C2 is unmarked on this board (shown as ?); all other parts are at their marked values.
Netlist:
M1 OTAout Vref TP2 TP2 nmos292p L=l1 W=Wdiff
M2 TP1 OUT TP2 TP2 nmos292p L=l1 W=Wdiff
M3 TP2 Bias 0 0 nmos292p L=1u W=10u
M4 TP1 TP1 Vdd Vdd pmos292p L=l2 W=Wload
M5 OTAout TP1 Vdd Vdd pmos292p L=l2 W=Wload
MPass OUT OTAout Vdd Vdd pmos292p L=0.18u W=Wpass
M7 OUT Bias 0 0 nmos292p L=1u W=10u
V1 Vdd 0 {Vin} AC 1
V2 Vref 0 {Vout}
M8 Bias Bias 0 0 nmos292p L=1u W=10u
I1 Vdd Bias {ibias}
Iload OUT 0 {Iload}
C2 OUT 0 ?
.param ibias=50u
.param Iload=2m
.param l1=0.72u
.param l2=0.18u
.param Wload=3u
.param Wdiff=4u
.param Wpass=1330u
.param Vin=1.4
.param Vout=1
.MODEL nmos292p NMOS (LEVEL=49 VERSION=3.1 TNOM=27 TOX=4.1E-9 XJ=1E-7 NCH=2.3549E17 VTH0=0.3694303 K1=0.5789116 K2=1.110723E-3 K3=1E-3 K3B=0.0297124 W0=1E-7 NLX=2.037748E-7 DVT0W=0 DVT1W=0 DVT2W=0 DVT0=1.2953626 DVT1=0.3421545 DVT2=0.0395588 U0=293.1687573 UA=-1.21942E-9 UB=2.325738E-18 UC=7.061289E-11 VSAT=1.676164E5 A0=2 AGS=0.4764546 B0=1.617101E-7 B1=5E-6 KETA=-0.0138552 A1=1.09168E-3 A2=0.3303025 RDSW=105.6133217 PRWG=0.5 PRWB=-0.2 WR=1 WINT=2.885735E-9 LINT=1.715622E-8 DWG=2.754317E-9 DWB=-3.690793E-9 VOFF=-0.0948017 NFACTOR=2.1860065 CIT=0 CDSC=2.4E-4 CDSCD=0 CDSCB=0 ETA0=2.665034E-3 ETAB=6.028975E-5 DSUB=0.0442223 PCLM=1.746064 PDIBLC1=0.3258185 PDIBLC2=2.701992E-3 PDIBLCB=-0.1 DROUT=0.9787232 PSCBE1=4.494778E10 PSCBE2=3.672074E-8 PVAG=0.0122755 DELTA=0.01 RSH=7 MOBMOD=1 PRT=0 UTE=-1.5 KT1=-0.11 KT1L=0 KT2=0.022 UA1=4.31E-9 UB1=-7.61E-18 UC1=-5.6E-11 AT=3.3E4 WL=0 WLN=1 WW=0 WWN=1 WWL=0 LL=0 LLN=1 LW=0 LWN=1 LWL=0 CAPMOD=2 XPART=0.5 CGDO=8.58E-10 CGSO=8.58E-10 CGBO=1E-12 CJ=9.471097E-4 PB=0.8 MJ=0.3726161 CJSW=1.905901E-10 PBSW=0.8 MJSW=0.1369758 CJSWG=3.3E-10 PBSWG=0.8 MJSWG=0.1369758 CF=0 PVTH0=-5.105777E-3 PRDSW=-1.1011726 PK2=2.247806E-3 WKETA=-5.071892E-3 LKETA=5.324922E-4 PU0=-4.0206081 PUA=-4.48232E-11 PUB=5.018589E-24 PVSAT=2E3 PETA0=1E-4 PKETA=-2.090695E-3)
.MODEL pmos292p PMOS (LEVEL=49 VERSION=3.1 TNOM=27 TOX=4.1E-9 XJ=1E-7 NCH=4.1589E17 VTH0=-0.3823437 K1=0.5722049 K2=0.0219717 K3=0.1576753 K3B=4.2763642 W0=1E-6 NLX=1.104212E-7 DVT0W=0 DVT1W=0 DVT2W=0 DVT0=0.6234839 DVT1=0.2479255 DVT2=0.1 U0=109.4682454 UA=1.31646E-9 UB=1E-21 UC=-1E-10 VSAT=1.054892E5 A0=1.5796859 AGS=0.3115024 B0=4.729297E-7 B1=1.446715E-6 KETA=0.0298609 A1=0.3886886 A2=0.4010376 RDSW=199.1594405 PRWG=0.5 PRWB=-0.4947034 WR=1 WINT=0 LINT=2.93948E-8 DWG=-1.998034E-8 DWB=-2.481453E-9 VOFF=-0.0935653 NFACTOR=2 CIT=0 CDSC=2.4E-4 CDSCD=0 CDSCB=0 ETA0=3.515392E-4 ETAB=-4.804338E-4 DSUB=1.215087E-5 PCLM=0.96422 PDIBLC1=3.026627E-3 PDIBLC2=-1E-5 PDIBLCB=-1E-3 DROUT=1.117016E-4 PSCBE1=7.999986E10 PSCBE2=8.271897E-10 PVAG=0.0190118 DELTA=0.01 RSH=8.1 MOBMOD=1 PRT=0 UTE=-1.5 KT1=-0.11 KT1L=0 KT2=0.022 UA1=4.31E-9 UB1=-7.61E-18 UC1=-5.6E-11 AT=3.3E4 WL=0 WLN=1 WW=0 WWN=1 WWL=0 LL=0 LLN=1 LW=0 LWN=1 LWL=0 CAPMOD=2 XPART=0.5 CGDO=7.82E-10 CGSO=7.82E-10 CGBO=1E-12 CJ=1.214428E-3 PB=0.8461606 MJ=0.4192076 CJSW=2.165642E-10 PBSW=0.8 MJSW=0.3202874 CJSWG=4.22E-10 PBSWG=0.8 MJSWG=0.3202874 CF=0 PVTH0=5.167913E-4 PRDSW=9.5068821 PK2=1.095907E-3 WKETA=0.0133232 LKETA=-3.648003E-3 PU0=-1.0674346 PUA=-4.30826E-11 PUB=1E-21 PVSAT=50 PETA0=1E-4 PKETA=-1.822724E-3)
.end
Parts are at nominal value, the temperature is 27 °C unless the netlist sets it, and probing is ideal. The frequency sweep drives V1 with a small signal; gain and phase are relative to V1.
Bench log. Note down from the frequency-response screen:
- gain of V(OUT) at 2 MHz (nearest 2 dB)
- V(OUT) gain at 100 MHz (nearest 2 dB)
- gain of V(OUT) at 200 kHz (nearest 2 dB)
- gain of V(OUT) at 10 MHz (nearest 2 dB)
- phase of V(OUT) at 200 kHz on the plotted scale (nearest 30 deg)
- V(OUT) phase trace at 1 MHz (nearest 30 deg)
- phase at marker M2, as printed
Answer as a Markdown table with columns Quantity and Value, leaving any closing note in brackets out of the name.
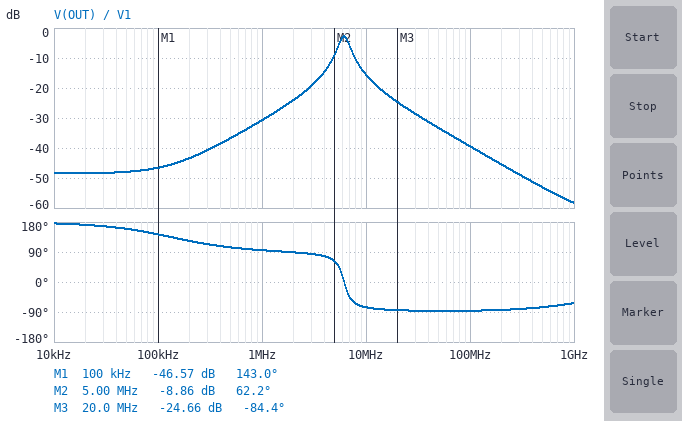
| Quantity | Value |
|---|---|
| gain of V(OUT) at 2 MHz | -24 dB |
| V(OUT) gain at 100 MHz | -40 dB |
| gain of V(OUT) at 200 kHz | -44 dB |
| gain of V(OUT) at 10 MHz | -16 dB |
| phase of V(OUT) at 200 kHz on the plotted scale | 120 deg |
| V(OUT) phase trace at 1 MHz | 90 deg |
| phase at marker M2, as printed | 62.2 deg |
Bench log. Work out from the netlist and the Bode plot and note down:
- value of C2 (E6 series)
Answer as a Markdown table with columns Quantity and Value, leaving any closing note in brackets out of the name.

| Quantity | Value |
|---|---|
| value of C2 | 1.5 nF |
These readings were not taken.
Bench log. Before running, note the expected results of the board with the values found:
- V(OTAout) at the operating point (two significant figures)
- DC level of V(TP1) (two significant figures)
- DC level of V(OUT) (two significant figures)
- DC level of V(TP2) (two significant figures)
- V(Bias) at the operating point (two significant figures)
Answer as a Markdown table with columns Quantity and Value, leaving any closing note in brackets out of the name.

| Quantity | Value |
|---|---|
| V(OTAout) at the operating point | 840 mV |
| DC level of V(TP1) | 750 mV |
| DC level of V(OUT) | 1.0 V |
| DC level of V(TP2) | 380 mV |
| V(Bias) at the operating point | 620 mV |
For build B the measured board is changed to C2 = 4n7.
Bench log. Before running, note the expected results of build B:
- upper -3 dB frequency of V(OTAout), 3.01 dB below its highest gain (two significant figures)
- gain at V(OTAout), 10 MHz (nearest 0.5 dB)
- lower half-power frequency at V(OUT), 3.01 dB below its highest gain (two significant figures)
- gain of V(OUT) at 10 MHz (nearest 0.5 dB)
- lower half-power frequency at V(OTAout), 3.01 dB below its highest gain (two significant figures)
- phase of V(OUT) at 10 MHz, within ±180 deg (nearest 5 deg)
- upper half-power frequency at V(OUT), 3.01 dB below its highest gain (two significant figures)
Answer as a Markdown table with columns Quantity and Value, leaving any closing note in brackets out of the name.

| Quantity | Value |
|---|---|
| upper -3 dB frequency of V(OTAout), 3.01 dB below its highest gain | 3.7 MHz |
| gain at V(OTAout), 10 MHz | -4.5 dB |
| lower half-power frequency at V(OUT), 3.01 dB below its highest gain | 3.1 MHz |
| gain of V(OUT) at 10 MHz | -28.5 dB |
| lower half-power frequency at V(OTAout), 3.01 dB below its highest gain | 2.7 MHz |
| phase of V(OUT) at 10 MHz, within ±180 deg | -85 deg |
| upper half-power frequency at V(OUT), 3.01 dB below its highest gain | 3.9 MHz |
